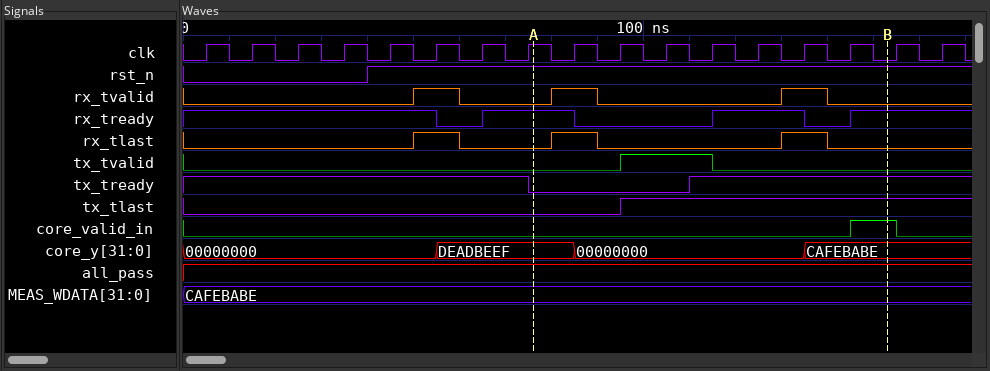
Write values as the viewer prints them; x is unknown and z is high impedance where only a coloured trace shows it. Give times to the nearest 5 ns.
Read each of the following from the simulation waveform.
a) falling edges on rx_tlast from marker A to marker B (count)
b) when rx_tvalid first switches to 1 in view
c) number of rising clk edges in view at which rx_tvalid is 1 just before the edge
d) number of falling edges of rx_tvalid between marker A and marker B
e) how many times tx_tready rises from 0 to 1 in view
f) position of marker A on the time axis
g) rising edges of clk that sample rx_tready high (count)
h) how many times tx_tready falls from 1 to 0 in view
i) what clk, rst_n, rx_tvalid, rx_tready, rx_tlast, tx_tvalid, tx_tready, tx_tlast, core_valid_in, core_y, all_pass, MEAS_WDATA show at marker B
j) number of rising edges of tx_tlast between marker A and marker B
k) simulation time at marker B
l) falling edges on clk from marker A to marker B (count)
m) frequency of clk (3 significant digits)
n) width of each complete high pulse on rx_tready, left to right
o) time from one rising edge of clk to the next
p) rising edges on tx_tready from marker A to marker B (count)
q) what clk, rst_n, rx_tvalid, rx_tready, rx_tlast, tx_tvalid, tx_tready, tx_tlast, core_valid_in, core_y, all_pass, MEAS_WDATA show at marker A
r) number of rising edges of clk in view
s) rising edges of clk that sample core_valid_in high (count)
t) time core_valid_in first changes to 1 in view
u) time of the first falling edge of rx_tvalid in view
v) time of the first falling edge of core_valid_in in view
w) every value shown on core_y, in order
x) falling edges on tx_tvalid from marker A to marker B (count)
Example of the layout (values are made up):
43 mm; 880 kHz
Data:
2; 50 ns; 3; 2; 1; 75 ns; 12; 1; clk=0, rst_n=1, rx_tvalid=0, rx_tready=1, rx_tlast=0, tx_tvalid=0, tx_tready=1, tx_tlast=1, core_valid_in=1, core_y=CAFEBABE, all_pass=1, MEAS_WDATA=CAFEBABE; 1; 155 ns; 8; 100 MHz; 20 ns, 20 ns; 10 ns; 1; clk=1, rst_n=1, rx_tvalid=0, rx_tready=1, rx_tlast=0, tx_tvalid=0, tx_tready=0, tx_tlast=0, core_valid_in=0, core_y=DEADBEEF, all_pass=1, MEAS_WDATA=CAFEBABE; 17; 1; 145 ns; 60 ns; 155 ns; 00000000, DEADBEEF, 00000000, CAFEBABE; 1
